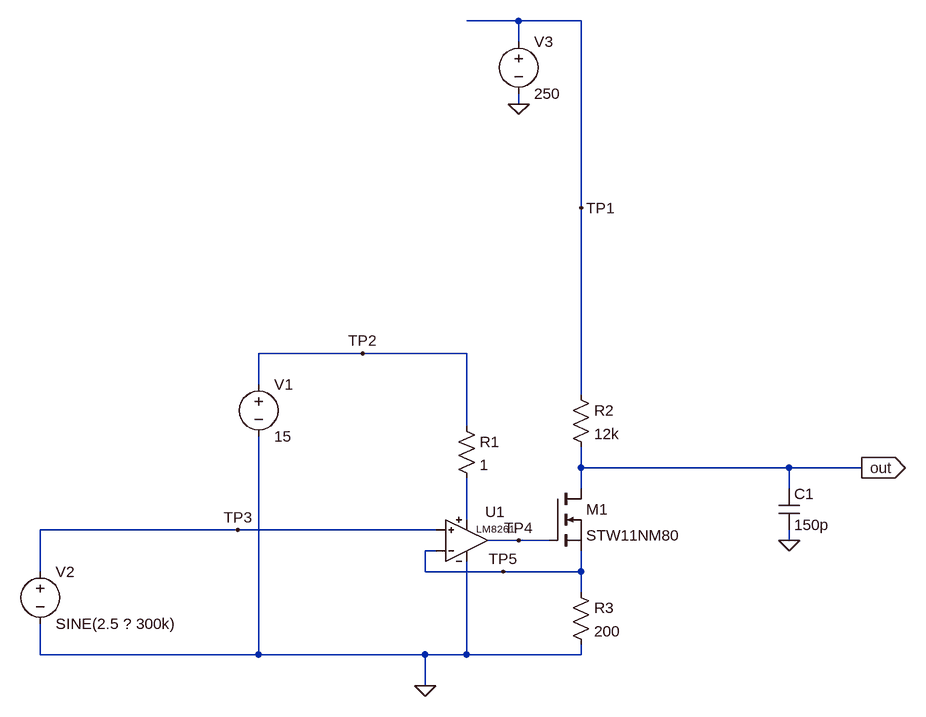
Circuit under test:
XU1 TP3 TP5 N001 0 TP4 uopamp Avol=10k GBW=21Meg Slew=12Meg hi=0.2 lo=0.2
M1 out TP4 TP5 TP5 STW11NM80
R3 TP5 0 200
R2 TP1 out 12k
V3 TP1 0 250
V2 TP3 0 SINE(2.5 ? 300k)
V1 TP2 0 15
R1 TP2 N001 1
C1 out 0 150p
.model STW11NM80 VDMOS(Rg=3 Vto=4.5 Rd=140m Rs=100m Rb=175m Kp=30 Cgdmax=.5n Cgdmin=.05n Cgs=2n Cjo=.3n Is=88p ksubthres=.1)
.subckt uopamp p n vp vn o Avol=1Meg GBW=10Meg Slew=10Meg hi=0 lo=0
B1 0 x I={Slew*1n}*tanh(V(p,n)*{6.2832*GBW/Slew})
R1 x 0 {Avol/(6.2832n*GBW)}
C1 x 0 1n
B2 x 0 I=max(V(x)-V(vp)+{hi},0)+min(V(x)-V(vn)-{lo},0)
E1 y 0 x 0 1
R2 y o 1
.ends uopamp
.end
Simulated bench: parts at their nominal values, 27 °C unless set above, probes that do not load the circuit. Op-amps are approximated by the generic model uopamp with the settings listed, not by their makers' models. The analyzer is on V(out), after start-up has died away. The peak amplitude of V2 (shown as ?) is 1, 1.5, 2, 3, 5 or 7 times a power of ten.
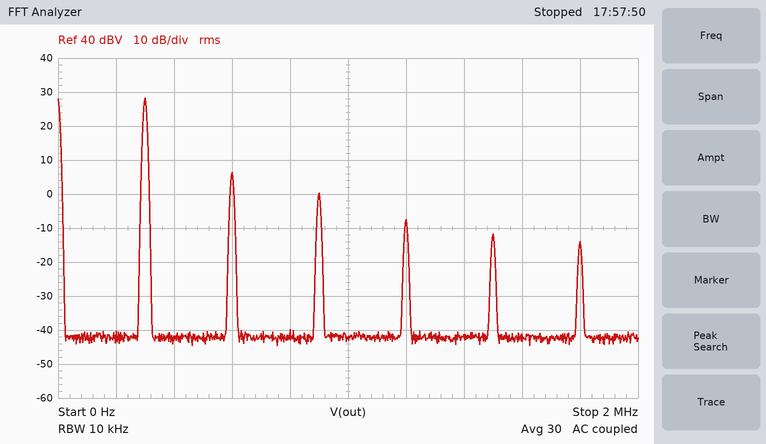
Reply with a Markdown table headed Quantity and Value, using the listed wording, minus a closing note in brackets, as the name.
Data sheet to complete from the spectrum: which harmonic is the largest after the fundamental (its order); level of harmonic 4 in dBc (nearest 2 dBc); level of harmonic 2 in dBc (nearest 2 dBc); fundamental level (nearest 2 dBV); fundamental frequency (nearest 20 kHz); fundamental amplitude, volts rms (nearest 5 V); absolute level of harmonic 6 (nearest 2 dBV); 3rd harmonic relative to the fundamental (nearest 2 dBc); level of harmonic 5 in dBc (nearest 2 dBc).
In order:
| Quantity | Value |
|---|---|
| which harmonic is the largest after the fundamental | 2 |
| level of harmonic 4 in dBc | -36 dBc |
| level of harmonic 2 in dBc | -22 dBc |
| fundamental level | 28 dBV |
| fundamental frequency | 300 kHz |
| fundamental amplitude, volts rms | 25 V |
| absolute level of harmonic 6 | -14 dBV |
| 3rd harmonic relative to the fundamental | -28 dBc |
| level of harmonic 5 in dBc | -40 dBc |
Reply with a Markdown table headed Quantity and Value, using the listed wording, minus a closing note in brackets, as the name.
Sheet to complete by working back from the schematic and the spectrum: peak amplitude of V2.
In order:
| Quantity | Value |
|---|---|
| peak amplitude of V2 | 3 V |
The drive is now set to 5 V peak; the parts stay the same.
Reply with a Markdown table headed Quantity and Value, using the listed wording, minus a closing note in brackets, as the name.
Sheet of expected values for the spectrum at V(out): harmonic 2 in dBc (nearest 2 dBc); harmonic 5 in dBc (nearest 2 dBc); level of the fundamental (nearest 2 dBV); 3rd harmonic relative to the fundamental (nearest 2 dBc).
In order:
| Quantity | Value |
|---|---|
| harmonic 2 in dBc | -12 dBc |
| harmonic 5 in dBc | -36 dBc |
| level of the fundamental | 30 dBV |
| 3rd harmonic relative to the fundamental | -26 dBc |
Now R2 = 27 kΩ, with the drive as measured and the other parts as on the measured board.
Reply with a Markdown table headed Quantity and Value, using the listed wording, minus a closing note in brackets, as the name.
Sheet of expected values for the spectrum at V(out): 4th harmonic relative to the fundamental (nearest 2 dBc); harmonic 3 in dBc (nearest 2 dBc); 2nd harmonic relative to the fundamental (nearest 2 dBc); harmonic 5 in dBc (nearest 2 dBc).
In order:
| Quantity | Value |
|---|---|
| 4th harmonic relative to the fundamental | -30 dBc |
| harmonic 3 in dBc | -20 dBc |
| 2nd harmonic relative to the fundamental | -10 dBc |
| harmonic 5 in dBc | -26 dBc |
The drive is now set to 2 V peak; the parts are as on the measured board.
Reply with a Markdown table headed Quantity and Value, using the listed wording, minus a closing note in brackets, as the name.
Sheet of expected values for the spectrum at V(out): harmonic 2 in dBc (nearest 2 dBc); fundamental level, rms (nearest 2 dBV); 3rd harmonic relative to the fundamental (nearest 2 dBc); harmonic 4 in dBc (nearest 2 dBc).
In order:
| Quantity | Value |
|---|---|
| harmonic 2 in dBc | -42 dBc |
| fundamental level, rms | 26 dBV |
| 3rd harmonic relative to the fundamental | -50 dBc |
| harmonic 4 in dBc | -56 dBc |
